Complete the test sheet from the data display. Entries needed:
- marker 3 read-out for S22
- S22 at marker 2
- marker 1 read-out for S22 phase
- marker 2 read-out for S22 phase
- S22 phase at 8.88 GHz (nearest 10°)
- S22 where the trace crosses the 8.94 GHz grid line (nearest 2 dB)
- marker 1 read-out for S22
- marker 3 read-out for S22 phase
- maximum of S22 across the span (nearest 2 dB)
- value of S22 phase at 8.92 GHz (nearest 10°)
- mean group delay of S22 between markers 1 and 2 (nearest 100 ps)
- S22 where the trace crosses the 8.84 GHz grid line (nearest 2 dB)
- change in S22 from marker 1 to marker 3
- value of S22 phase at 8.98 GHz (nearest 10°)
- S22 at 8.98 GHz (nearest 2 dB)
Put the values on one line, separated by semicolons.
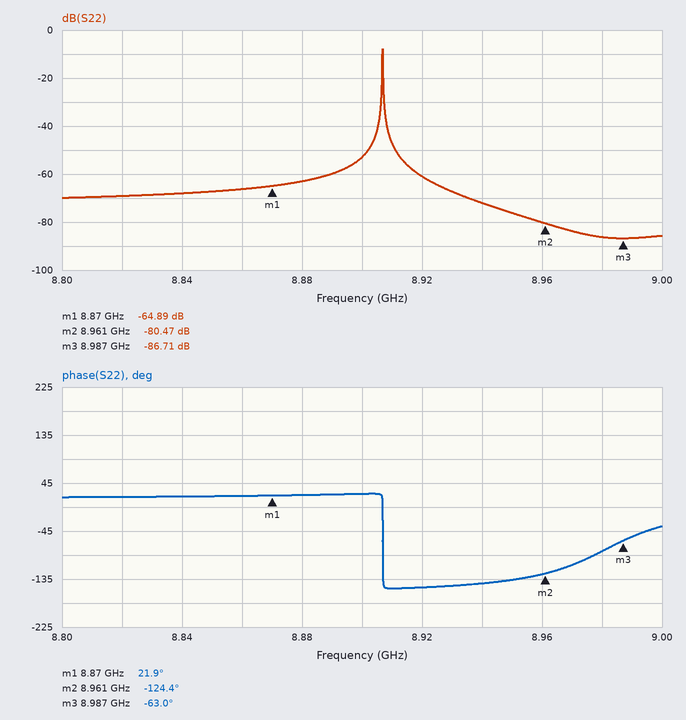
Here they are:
-86.71 dB; -80.47 dB; 21.9°; -124.4°; 20°; -72 dB; -64.89 dB; -63.0°; -8 dB; -150°; 4.5 ns; -68 dB; -21.82 dB; -80°; -86 dB
